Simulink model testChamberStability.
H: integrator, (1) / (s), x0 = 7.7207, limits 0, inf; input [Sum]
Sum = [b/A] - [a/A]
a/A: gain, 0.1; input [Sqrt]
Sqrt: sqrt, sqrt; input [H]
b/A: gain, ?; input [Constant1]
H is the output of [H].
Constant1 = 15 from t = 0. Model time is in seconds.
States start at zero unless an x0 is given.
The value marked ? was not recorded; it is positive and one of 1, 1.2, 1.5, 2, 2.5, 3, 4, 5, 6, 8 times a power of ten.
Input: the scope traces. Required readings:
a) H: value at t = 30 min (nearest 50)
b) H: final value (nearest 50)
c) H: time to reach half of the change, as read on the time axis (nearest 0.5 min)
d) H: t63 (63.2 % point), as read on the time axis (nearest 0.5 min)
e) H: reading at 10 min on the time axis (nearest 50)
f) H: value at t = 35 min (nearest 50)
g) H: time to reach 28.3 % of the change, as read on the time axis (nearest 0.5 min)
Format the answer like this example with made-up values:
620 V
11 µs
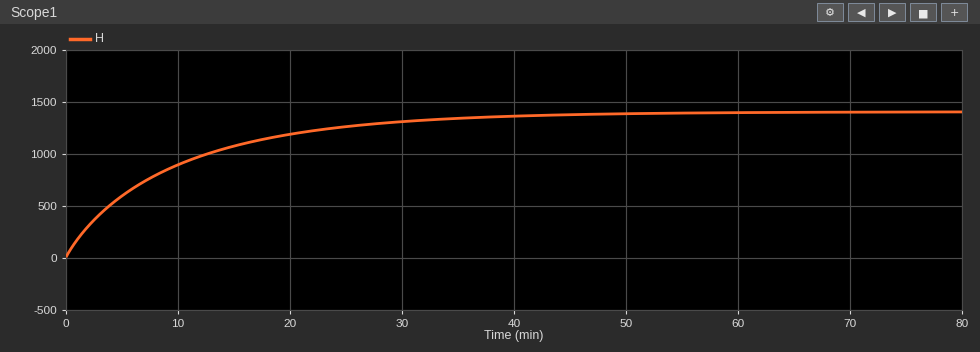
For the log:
1300
1400
6.5 min
10.0 min
900
1350
3.0 min
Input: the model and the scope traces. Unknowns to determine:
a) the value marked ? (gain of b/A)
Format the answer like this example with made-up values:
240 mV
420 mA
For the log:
0.25
